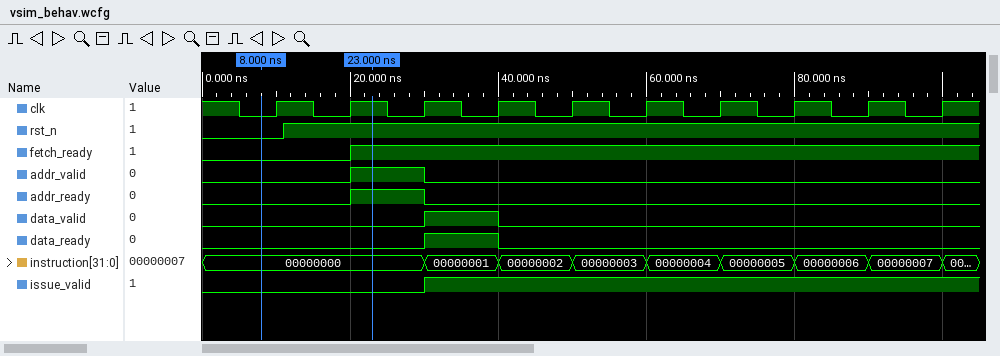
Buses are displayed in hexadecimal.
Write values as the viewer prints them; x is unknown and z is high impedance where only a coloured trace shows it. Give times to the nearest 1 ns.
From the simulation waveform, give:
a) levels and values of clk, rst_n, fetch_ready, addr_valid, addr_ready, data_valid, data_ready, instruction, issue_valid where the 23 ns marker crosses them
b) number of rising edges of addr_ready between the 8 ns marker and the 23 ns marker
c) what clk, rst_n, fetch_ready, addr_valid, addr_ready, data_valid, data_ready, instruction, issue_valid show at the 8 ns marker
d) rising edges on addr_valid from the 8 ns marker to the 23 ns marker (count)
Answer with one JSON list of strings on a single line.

["clk=1, rst_n=1, fetch_ready=1, addr_valid=1, addr_ready=1, data_valid=0, data_ready=0, instruction=00000000, issue_valid=0", "1", "clk=0, rst_n=0, fetch_ready=0, addr_valid=0, addr_ready=0, data_valid=0, data_ready=0, instruction=00000000, issue_valid=0", "1"]
